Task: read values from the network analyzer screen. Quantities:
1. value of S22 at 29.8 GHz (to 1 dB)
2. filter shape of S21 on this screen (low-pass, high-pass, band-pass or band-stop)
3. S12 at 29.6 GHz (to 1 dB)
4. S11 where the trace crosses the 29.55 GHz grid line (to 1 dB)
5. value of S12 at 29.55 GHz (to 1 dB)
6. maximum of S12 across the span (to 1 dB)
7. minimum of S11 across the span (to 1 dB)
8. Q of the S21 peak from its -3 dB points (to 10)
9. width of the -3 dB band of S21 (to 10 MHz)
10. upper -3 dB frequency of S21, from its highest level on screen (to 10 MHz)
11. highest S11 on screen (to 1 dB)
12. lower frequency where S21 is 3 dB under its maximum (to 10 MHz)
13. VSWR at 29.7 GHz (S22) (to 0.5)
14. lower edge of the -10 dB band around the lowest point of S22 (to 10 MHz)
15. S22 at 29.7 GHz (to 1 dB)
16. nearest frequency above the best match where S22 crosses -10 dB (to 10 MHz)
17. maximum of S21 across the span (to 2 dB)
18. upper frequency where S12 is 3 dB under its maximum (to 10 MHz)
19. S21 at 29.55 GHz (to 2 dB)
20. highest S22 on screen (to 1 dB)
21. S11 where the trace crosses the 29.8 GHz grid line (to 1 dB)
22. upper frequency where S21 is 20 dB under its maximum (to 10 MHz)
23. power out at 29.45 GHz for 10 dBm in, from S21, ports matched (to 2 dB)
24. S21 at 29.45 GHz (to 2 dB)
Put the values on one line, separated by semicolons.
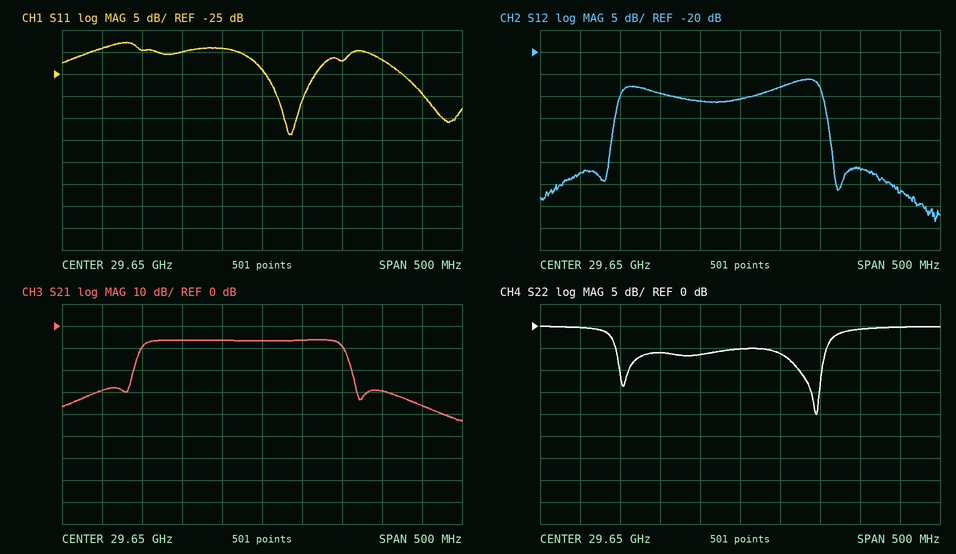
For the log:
-1 dB; band-pass; -31 dB; -20 dB; -29 dB; -26 dB; -39 dB; 120; 250 MHz; 29.75 GHz; -18 dB; 29.50 GHz; 3.0; 29.72 GHz; -6 dB; 29.75 GHz; -6 dB; 29.75 GHz; -6 dB; 0 dB; -22 dB; 29.77 GHz; -20 dBm; -30 dB
